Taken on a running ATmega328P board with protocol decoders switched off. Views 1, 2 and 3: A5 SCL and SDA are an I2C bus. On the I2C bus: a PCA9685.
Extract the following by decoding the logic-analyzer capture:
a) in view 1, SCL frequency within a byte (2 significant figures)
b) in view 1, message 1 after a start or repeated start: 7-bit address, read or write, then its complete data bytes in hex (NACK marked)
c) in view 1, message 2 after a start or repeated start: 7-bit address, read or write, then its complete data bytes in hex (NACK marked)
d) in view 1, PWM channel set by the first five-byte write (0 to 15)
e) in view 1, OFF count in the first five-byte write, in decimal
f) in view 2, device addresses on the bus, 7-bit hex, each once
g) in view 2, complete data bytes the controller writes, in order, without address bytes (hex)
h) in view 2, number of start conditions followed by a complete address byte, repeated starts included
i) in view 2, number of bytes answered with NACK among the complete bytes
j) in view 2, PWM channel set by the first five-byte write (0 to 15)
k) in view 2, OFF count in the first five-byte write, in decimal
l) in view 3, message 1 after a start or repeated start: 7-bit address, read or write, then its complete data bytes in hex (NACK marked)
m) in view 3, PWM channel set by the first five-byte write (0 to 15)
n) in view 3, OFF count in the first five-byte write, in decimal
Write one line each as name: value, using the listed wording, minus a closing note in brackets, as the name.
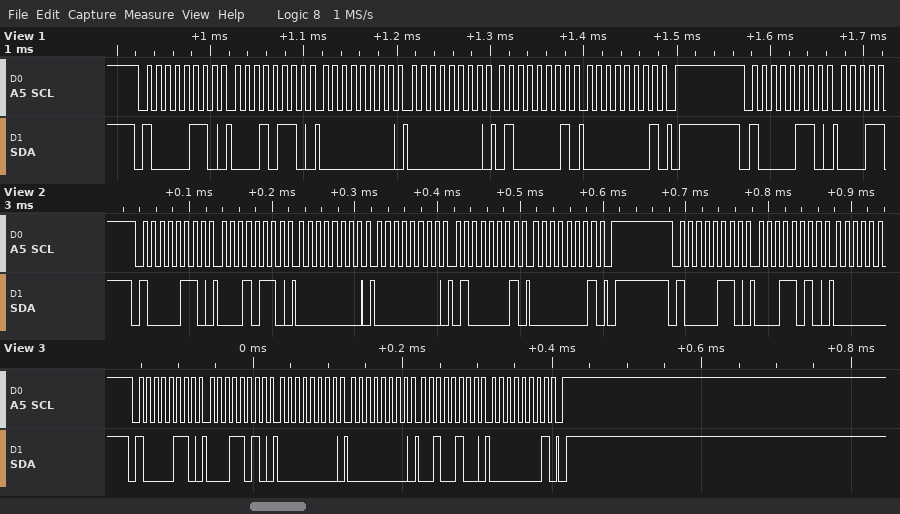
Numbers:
in view 1, SCL frequency within a byte: 100 kHz
in view 1, message 1 after a start or repeated start: 7-bit address, read or write, then its complete data bytes in hex: 0x43 write: 16 00 00 41 01
in view 1, message 2 after a start or repeated start: 7-bit address, read or write, then its complete data bytes in hex: 0x43 write
in view 1, PWM channel set by the first five-byte write: 4
in view 1, OFF count in the first five-byte write, in decimal: 321
in view 2, device addresses on the bus, 7-bit hex, each once: 0x43
in view 2, complete data bytes the controller writes, in order, without address bytes: 16 00 00 41 01 1A
in view 2, number of start conditions followed by a complete address byte, repeated starts included: 2
in view 2, number of bytes answered with NACK among the complete bytes: 0
in view 2, PWM channel set by the first five-byte write: 4
in view 2, OFF count in the first five-byte write, in decimal: 321
in view 3, message 1 after a start or repeated start: 7-bit address, read or write, then its complete data bytes in hex: 0x43 write: 1A 00 00 24 01
in view 3, PWM channel set by the first five-byte write: 5
in view 3, OFF count in the first five-byte write, in decimal: 292
